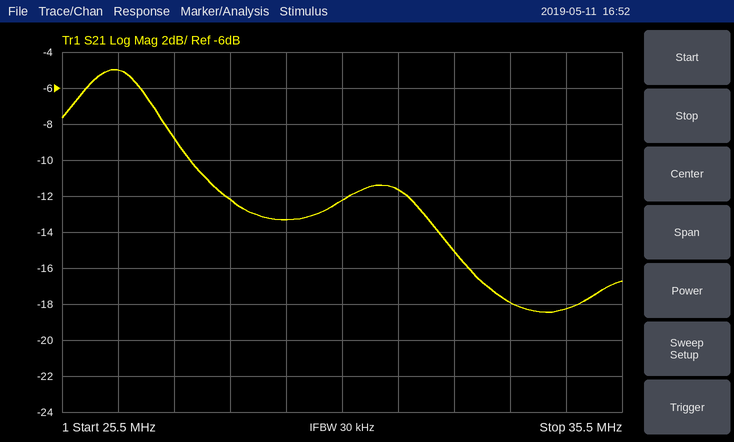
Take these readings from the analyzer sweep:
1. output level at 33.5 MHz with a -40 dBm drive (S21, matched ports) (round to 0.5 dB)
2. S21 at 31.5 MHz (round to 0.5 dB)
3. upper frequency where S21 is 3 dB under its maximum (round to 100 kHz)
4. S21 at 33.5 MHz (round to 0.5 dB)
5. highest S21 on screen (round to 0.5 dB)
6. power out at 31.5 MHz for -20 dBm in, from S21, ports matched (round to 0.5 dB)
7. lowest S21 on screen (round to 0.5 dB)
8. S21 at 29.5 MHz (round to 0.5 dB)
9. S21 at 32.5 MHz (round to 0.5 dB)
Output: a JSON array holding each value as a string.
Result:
["-58.0 dBm", "-11.5 dB", "27.3 MHz", "-18.0 dB", "-5.0 dB", "-31.5 dBm", "-18.5 dB", "-13.5 dB", "-15.0 dB"]
